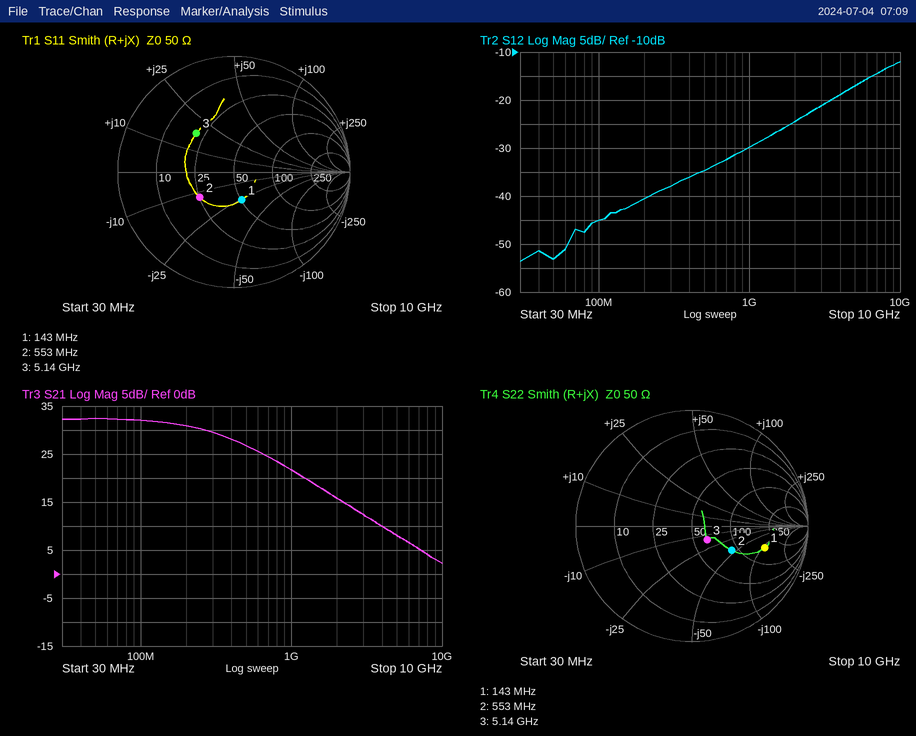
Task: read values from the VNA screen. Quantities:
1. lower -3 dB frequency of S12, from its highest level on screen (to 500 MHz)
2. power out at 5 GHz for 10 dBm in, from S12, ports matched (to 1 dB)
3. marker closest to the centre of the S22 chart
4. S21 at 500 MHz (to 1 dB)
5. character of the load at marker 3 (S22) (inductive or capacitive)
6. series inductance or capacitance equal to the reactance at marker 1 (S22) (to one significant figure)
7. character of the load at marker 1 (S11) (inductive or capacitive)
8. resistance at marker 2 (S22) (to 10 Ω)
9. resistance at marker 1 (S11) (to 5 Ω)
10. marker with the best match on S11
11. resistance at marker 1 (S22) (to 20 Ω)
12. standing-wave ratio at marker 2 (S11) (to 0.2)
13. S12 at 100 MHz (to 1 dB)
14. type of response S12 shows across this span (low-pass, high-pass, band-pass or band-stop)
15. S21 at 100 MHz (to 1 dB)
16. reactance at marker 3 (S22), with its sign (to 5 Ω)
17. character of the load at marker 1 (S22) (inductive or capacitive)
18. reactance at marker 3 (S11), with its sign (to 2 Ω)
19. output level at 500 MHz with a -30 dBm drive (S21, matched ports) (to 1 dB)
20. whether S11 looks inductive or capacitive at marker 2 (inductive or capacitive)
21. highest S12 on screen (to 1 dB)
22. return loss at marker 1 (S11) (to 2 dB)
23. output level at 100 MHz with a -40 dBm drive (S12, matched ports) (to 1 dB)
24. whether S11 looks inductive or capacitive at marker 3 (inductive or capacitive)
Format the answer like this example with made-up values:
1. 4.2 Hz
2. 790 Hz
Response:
1. 6.5 GHz
2. -7 dBm
3. marker 3
4. 27 dB
5. capacitive
6. 10 pF
7. capacitive
8. 90 Ω
9. 50 Ω
10. marker 1
11. 160 Ω
12. 2.2
13. -45 dB
14. high-pass
15. 32 dB
16. -15 Ω
17. capacitive
18. +18 Ω
19. -3 dBm
20. capacitive
21. -12 dB
22. 12 dB
23. -85 dBm
24. inductive
